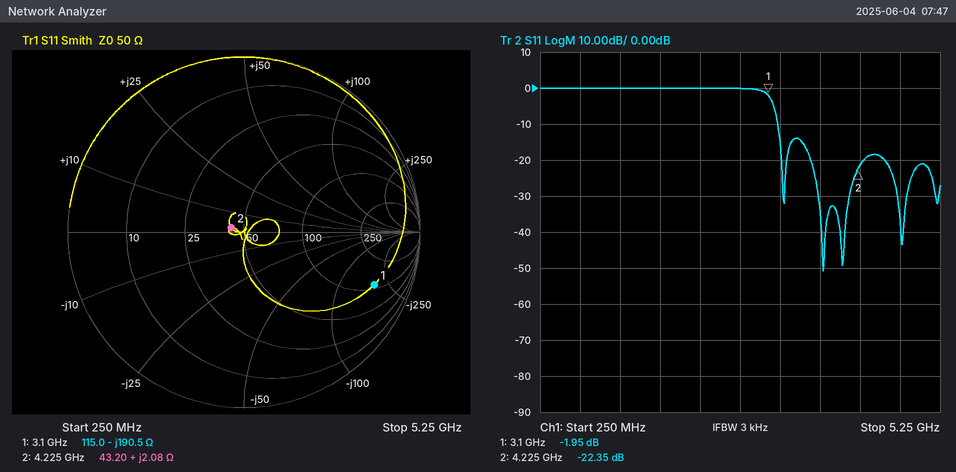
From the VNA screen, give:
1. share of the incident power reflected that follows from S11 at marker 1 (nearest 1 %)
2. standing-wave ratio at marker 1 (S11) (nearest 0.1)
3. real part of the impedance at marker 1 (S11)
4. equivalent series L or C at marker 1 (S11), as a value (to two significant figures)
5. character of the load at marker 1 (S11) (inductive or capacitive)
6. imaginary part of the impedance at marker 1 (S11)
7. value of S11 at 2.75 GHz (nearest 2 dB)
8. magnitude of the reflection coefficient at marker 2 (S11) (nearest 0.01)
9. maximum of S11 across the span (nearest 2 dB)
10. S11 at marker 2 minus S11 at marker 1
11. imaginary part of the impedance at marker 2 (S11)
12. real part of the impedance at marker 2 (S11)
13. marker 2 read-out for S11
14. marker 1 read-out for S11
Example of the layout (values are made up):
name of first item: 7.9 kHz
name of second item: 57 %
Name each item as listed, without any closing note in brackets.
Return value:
share of the incident power reflected that follows from S11 at marker 1: 64 %
standing-wave ratio at marker 1 (S11): 8.9
real part of the impedance at marker 1: 115.0 Ω
equivalent series L or C at marker 1 (S11), as a value: 270 fF
character of the load at marker 1 (S11): capacitive
imaginary part of the impedance at marker 1: -190.5 Ω
value of S11 at 2.75 GHz: 0 dB
magnitude of the reflection coefficient at marker 2 (S11): 0.08
maximum of S11 across the span: 0 dB
S11 at marker 2 minus S11 at marker 1: -20.40 dB
imaginary part of the impedance at marker 2: +2.08 Ω
real part of the impedance at marker 2: 43.20 Ω
marker 2 read-out for S11: -22.35 dB
marker 1 read-out for S11: -1.95 dB
